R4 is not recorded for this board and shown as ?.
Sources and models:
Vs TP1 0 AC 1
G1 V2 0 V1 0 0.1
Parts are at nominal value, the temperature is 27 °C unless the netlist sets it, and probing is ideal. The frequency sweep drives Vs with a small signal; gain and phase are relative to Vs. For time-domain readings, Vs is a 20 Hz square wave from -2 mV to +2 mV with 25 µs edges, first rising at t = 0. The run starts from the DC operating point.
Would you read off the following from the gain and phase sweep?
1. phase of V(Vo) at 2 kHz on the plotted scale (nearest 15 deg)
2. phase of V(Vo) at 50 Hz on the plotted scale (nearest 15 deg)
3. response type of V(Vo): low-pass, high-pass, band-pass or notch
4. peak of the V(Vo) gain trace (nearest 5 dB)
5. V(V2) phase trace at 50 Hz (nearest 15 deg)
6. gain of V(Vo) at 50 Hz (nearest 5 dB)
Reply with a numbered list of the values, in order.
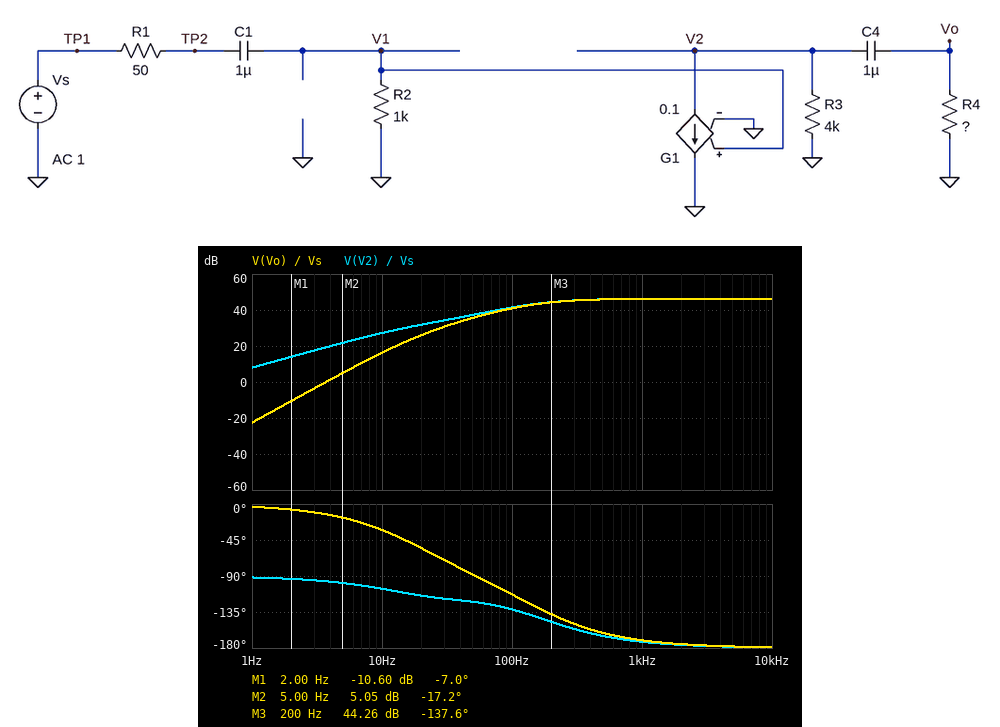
1. -180 deg
2. -90 deg
3. high-pass
4. 45 dB
5. -120 deg
6. 35 dB
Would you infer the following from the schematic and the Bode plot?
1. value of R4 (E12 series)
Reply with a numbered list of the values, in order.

1. 4.7 kΩ
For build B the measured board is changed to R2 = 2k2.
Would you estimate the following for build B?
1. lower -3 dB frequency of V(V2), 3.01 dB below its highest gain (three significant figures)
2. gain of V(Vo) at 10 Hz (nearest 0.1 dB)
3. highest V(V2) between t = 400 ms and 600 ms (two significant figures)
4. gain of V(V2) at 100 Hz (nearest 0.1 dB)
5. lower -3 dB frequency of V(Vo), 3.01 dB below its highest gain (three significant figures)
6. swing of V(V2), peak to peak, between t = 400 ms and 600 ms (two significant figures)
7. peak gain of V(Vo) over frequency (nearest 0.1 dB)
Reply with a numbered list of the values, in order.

1. 59.3 Hz
2. 23.0 dB
3. 830 mV
4. 45.1 dB
5. 75.1 Hz
6. 1.7 V
7. 46.5 dB
